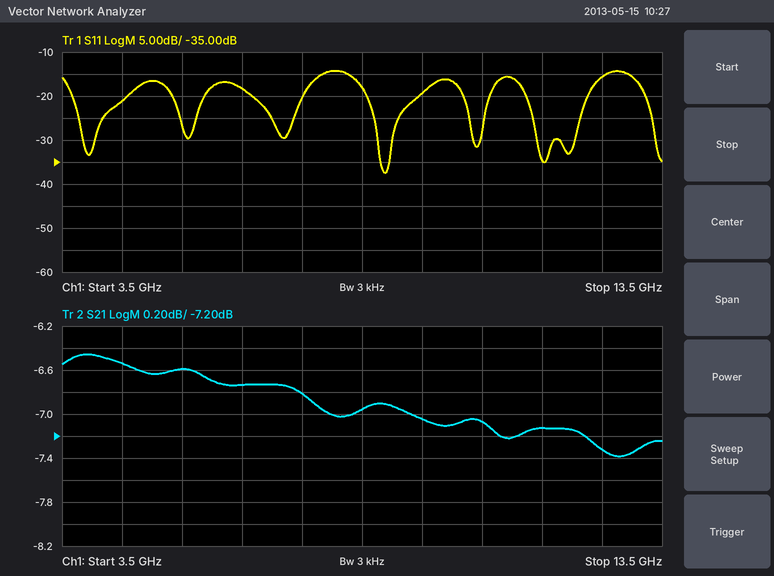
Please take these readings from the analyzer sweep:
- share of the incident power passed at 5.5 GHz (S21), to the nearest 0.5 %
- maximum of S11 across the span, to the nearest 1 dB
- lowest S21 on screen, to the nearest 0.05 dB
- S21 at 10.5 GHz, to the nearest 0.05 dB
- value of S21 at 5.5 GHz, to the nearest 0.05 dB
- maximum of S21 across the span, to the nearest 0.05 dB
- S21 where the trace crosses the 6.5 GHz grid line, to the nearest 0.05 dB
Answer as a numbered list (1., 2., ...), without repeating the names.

1. 22.0 %
2. -14 dB
3. -7.40 dB
4. -7.05 dB
5. -6.60 dB
6. -6.45 dB
7. -6.75 dB
